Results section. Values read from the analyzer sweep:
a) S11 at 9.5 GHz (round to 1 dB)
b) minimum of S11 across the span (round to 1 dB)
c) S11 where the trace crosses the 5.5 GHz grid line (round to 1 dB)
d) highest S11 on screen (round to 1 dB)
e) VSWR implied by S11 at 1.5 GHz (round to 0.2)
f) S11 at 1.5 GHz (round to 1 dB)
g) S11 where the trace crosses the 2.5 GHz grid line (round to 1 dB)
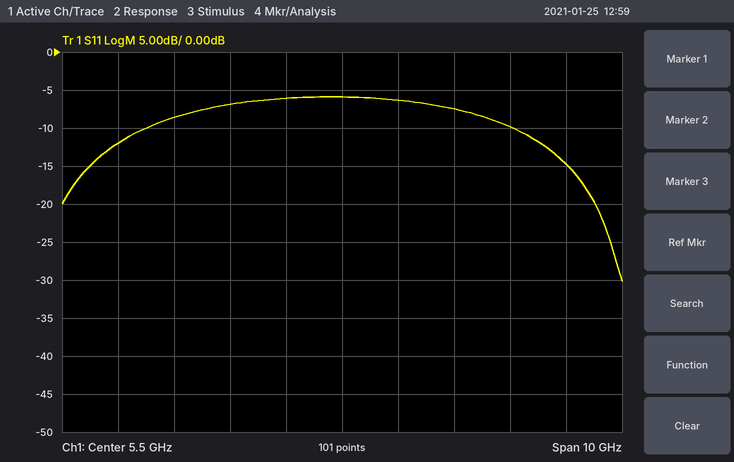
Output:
-15 dB
-30 dB
-6 dB
-6 dB
1.6
-12 dB
-9 dB
